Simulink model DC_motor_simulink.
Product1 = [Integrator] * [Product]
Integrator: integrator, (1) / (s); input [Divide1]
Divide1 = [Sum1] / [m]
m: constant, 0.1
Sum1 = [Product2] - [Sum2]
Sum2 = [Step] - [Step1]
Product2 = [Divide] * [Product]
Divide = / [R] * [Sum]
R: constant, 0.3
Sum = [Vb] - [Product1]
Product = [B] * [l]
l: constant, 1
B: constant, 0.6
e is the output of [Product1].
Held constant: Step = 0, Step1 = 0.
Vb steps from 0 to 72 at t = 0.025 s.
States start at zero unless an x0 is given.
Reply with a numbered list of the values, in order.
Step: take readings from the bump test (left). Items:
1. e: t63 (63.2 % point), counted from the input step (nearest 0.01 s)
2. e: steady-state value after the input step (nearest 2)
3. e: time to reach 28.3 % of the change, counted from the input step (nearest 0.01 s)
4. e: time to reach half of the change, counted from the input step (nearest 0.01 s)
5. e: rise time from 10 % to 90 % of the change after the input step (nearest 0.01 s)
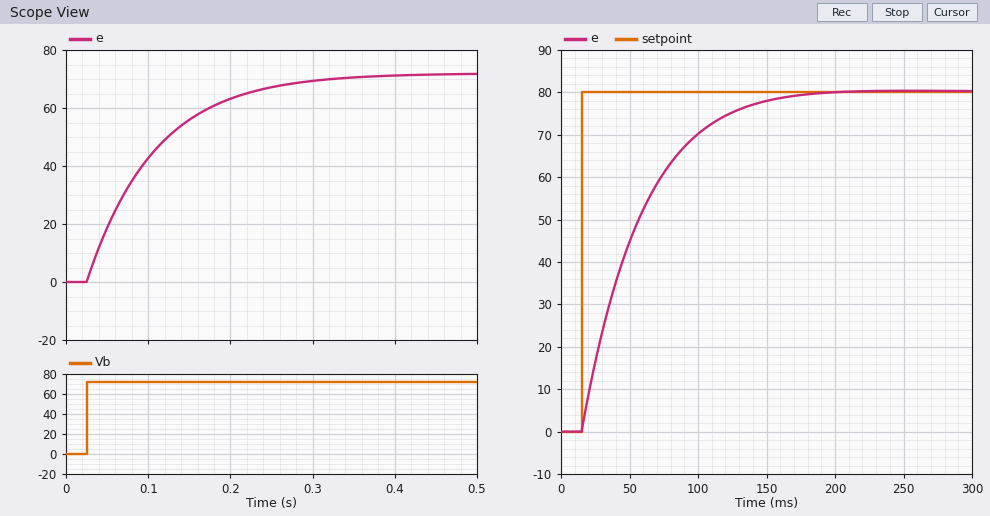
1. 0.08 s
2. 72
3. 0.03 s
4. 0.06 s
5. 0.18 s
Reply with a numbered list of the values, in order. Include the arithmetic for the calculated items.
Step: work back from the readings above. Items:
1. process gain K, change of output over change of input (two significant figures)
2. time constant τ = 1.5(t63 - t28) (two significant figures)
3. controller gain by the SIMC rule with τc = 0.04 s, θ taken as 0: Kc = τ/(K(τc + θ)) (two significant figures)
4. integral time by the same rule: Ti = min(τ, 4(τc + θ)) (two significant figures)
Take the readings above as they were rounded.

1. (72 - 0) / 72 = 1.0
2. 1.5 × (0.08 - 0.03) = 0.075 s
3. 0.075 / (1 × (0.04 + 0)) = 1.9
4. min(0.075, 4 × (0.04 + 0)) = 0.075 s
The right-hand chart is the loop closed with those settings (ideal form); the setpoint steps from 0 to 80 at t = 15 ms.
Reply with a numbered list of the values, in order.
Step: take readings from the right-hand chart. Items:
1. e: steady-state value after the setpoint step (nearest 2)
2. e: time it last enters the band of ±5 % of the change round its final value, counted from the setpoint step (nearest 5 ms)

1. 80
2. 115 ms
